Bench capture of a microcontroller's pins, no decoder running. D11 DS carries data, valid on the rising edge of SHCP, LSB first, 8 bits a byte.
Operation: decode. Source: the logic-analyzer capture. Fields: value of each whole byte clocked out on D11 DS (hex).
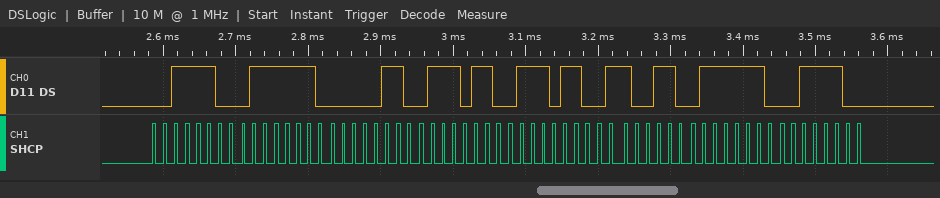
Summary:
3C 7E 60 6E 6E 66 7E 3C
